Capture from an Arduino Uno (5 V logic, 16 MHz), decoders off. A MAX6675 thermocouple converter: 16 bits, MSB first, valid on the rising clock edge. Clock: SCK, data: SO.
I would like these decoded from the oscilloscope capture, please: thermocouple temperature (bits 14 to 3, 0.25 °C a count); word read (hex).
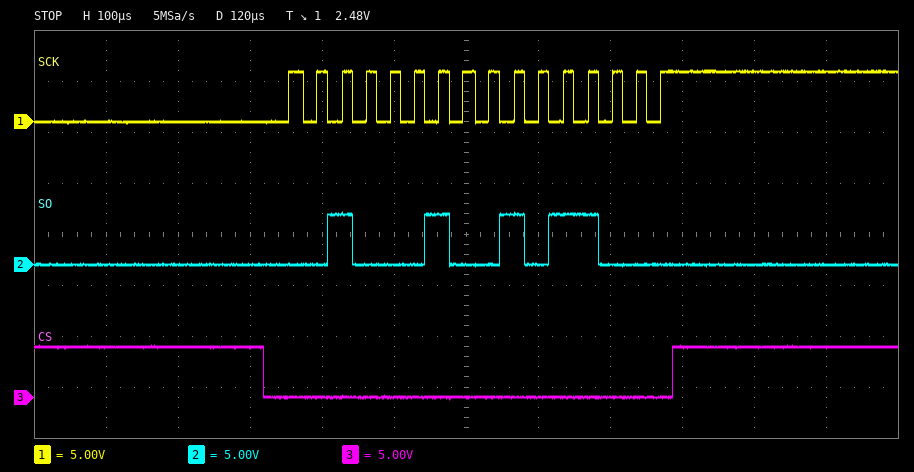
274.75 °C
0x2258
